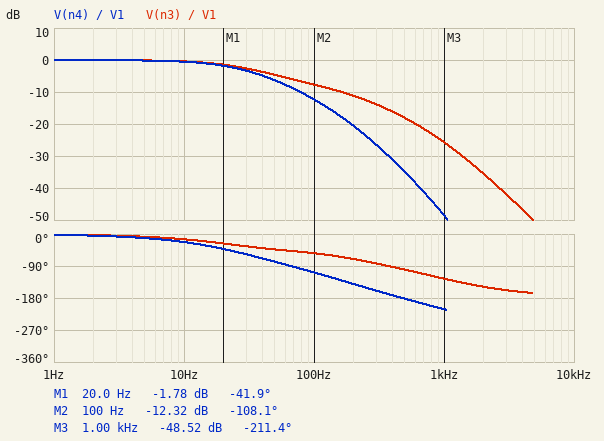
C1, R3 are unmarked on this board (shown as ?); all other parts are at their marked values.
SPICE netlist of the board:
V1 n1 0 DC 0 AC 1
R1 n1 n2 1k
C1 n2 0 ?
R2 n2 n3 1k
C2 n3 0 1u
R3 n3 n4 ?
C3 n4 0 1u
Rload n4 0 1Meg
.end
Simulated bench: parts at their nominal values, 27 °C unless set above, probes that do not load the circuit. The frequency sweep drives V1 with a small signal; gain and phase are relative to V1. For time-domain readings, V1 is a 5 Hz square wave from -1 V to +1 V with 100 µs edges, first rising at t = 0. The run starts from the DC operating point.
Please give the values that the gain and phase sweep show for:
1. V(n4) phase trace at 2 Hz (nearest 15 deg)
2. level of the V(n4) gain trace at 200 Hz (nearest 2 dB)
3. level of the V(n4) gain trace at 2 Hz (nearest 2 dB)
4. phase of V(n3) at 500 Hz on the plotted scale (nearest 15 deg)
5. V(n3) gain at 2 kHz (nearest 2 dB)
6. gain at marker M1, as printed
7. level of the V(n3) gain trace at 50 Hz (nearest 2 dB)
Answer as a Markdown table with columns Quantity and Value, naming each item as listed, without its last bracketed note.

| Quantity | Value |
|---|---|
| V(n4) phase trace at 2 Hz | 0 deg |
| level of the V(n4) gain trace at 200 Hz | -20 dB |
| level of the V(n4) gain trace at 2 Hz | 0 dB |
| phase of V(n3) at 500 Hz on the plotted scale | -105 deg |
| V(n3) gain at 2 kHz | -36 dB |
| gain at marker M1, as printed | -1.78 dB |
| level of the V(n3) gain trace at 50 Hz | -4 dB |
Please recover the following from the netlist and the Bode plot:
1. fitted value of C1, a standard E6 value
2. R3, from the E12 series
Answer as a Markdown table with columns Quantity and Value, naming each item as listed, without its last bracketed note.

| Quantity | Value |
|---|---|
| fitted value of C1, a standard E6 value | 330 nF |
| R3, from the E12 series | 2.2 kΩ |
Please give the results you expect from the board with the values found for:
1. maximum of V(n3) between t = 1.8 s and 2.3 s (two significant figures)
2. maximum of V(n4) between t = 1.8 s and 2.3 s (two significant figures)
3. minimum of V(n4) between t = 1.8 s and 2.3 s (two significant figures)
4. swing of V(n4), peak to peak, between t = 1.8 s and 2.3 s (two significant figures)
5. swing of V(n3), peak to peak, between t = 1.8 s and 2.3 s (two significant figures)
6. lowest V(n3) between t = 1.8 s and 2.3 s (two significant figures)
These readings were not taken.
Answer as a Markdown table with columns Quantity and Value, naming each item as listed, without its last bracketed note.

| Quantity | Value |
|---|---|
| maximum of V(n3) between t = 1.8 s and 2.3 s | 1.0 V |
| maximum of V(n4) between t = 1.8 s and 2.3 s | 1.0 V |
| minimum of V(n4) between t = 1.8 s and 2.3 s | -1.0 V |
| swing of V(n4), peak to peak, between t = 1.8 s and 2.3 s | 2.0 V |
| swing of V(n3), peak to peak, between t = 1.8 s and 2.3 s | 2.0 V |
| lowest V(n3) between t = 1.8 s and 2.3 s | -1.0 V |
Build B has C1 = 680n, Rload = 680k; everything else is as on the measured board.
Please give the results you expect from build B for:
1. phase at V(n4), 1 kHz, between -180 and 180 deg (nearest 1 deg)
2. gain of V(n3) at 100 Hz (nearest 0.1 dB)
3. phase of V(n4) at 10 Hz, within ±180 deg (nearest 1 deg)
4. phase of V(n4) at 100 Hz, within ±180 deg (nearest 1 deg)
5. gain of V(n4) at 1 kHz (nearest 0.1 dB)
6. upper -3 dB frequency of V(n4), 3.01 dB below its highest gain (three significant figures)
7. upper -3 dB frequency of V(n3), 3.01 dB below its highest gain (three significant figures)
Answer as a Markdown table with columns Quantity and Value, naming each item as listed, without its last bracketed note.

| Quantity | Value |
|---|---|
| phase at V(n4), 1 kHz, between -180 and 180 deg | 131 deg |
| gain of V(n3) at 100 Hz | -8.2 dB |
| phase of V(n4) at 10 Hz, within ±180 deg | -24 deg |
| phase of V(n4) at 100 Hz, within ±180 deg | -115 deg |
| gain of V(n4) at 1 kHz | -52.8 dB |
| upper -3 dB frequency of V(n4), 3.01 dB below its highest gain | 27.5 Hz |
| upper -3 dB frequency of V(n3), 3.01 dB below its highest gain | 32.4 Hz |
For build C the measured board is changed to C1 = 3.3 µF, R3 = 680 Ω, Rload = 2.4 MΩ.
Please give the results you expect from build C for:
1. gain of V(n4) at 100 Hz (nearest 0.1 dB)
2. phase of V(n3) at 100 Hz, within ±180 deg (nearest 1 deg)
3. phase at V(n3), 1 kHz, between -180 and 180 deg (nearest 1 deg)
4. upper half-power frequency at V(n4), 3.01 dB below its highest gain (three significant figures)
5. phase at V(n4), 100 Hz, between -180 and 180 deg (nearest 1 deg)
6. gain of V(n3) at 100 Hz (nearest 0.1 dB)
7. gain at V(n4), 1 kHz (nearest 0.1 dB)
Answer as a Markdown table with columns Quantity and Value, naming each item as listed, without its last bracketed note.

| Quantity | Value |
|---|---|
| gain of V(n4) at 100 Hz | -14.6 dB |
| phase of V(n3) at 100 Hz, within ±180 deg | -101 deg |
| phase at V(n3), 1 kHz, between -180 and 180 deg | -155 deg |
| upper half-power frequency at V(n4), 3.01 dB below its highest gain | 23.8 Hz |
| phase at V(n4), 100 Hz, between -180 and 180 deg | -124 deg |
| gain of V(n3) at 100 Hz | -13.9 dB |
| gain at V(n4), 1 kHz | -56.2 dB |
